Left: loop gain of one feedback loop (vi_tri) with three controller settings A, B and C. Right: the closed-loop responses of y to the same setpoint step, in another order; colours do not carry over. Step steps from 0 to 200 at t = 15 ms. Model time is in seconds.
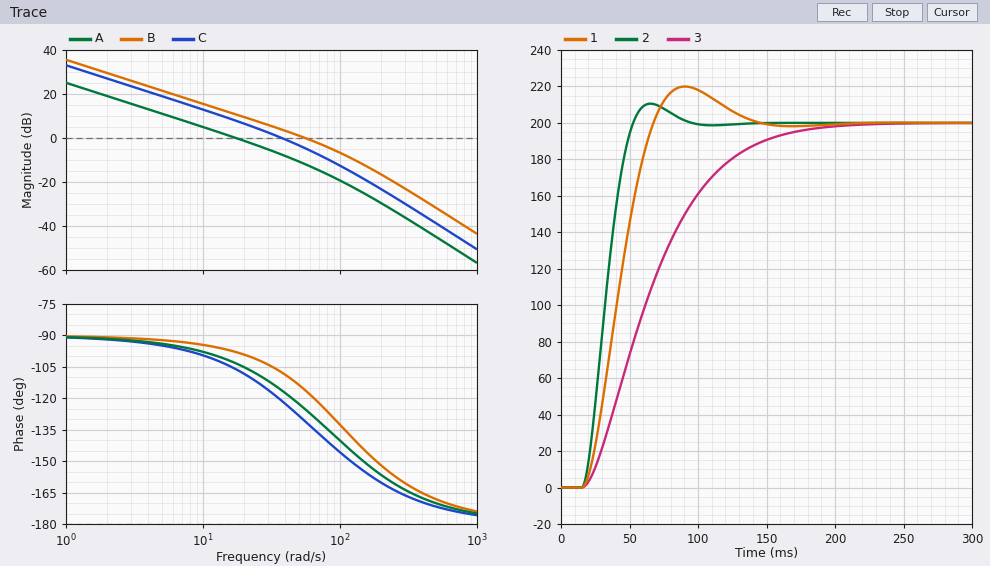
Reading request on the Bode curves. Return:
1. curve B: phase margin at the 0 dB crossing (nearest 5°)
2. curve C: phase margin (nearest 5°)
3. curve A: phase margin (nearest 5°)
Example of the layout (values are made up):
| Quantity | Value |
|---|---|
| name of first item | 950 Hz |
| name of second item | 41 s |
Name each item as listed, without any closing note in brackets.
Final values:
| Quantity | Value |
|---|---|
| curve B: phase margin at the 0 dB crossing | 65° |
| curve C: phase margin | 60° |
| curve A: phase margin | 75° |
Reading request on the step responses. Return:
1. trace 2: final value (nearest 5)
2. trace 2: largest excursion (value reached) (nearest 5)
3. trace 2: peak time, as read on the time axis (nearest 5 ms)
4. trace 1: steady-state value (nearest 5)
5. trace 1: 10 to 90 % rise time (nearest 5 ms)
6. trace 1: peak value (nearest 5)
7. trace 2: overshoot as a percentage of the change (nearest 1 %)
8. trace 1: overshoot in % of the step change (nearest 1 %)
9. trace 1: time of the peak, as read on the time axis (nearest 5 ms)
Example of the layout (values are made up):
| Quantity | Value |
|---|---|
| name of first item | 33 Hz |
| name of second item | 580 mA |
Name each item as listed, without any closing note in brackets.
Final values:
| Quantity | Value |
|---|---|
| trace 2: final value | 200 |
| trace 2: largest excursion (value reached) | 210 |
| trace 2: peak time, as read on the time axis | 65 ms |
| trace 1: steady-state value | 200 |
| trace 1: 10 to 90 % rise time | 35 ms |
| trace 1: peak value | 220 |
| trace 2: overshoot as a percentage of the change | 5 % |
| trace 1: overshoot in % of the step change | 10 % |
| trace 1: time of the peak, as read on the time axis | 90 ms |
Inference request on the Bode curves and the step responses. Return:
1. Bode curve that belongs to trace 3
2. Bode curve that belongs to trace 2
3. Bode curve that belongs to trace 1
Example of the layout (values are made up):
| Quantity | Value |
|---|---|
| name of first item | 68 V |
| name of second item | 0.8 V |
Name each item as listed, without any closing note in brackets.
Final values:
| Quantity | Value |
|---|---|
| Bode curve that belongs to trace 3 | A |
| Bode curve that belongs to trace 2 | B |
| Bode curve that belongs to trace 1 | C |
